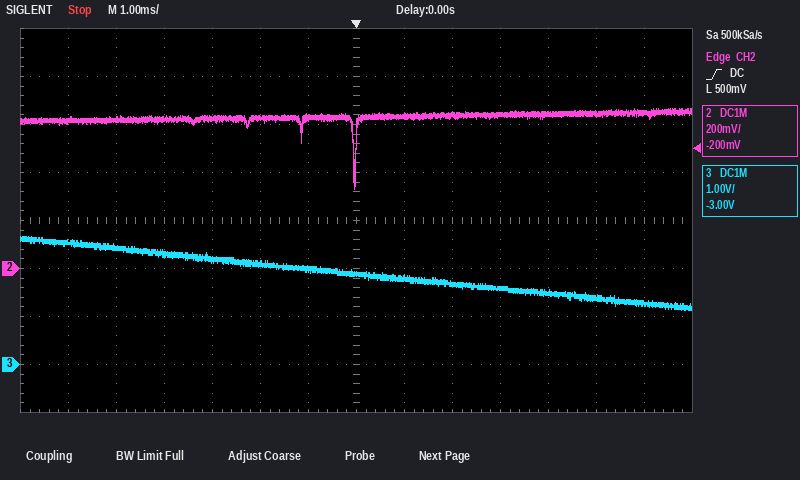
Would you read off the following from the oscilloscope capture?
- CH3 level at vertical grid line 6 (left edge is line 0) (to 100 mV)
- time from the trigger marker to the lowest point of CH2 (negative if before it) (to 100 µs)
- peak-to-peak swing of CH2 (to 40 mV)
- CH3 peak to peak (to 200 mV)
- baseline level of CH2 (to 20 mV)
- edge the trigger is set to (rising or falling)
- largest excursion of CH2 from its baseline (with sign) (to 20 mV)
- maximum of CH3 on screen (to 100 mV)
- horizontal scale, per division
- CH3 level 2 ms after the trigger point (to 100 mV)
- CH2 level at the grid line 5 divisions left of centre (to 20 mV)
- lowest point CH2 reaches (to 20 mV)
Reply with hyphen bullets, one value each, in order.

- 2.0 V
- 0.0 ms
- 320 mV
- 1.6 V
- 640 mV
- rising
- -300 mV
- 2.7 V
- 1 ms
- 1.7 V
- 620 mV
- 340 mV
